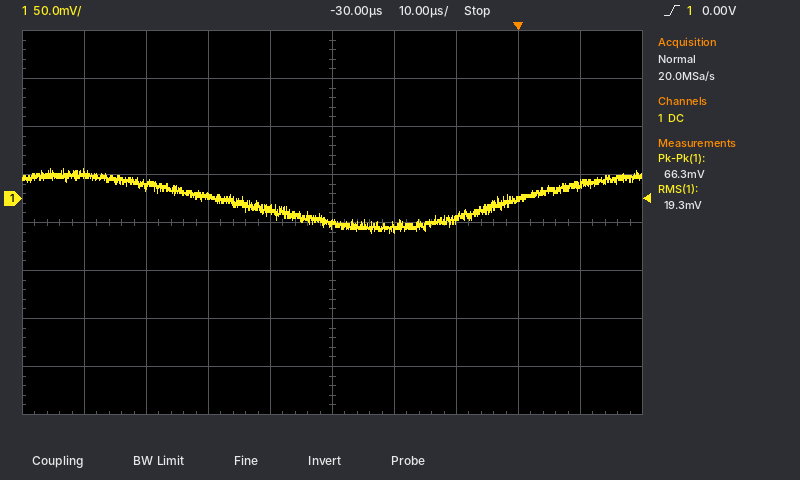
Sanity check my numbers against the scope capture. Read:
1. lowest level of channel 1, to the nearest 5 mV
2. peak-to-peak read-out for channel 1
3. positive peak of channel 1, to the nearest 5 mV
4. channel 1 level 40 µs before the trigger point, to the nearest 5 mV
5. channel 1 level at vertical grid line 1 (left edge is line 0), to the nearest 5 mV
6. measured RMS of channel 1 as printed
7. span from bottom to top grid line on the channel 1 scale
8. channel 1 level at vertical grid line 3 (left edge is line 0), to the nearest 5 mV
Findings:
-35 mV
66.3 mV
30 mV
-10 mV
25 mV
19.3 mV
400 mV
5 mV
